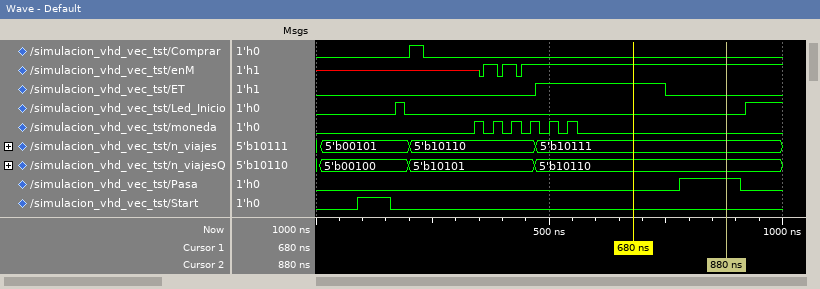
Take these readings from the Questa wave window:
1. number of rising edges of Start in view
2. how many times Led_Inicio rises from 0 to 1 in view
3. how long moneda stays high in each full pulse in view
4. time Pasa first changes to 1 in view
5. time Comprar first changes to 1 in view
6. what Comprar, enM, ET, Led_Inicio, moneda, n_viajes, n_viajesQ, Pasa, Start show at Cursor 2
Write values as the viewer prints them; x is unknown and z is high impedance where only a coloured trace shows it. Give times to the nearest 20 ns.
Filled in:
1
2
20 ns, 20 ns, 20 ns, 20 ns, 20 ns, 20 ns
780 ns
200 ns
Comprar=0, enM=1, ET=0, Led_Inicio=0, moneda=0, n_viajes=5'b10111, n_viajesQ=5'b10110, Pasa=1, Start=0
